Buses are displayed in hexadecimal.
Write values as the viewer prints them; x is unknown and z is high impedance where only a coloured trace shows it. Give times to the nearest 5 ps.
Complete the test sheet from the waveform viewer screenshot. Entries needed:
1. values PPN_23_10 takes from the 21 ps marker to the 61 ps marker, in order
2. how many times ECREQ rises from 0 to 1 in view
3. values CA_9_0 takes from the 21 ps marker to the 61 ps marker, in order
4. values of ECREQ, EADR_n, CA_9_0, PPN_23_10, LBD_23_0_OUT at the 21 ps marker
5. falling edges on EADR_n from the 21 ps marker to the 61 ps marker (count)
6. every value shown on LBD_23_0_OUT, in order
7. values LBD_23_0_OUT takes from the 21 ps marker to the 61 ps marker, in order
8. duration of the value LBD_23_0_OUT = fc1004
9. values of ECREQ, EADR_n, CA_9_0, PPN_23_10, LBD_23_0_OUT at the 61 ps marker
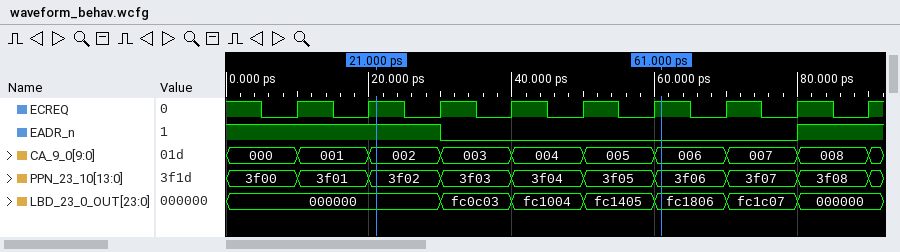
3f02, 3f03, 3f04, 3f05, 3f06
9
002, 003, 004, 005, 006
ECREQ=1, EADR_n=1, CA_9_0=002, PPN_23_10=3f02, LBD_23_0_OUT=000000
1
000000, fc0c03, fc1004, fc1405, fc1806, fc1c07, 000000
000000, fc0c03, fc1004, fc1405, fc1806
10 ps
ECREQ=1, EADR_n=0, CA_9_0=006, PPN_23_10=3f06, LBD_23_0_OUT=fc1806
